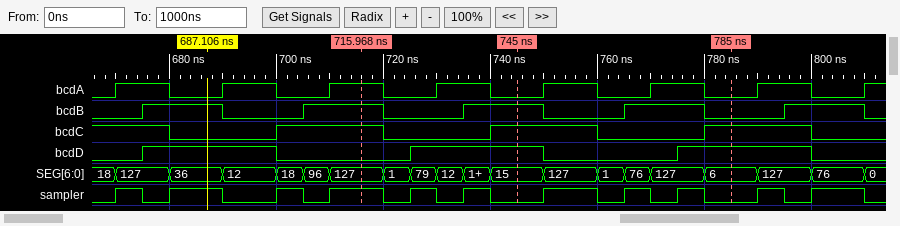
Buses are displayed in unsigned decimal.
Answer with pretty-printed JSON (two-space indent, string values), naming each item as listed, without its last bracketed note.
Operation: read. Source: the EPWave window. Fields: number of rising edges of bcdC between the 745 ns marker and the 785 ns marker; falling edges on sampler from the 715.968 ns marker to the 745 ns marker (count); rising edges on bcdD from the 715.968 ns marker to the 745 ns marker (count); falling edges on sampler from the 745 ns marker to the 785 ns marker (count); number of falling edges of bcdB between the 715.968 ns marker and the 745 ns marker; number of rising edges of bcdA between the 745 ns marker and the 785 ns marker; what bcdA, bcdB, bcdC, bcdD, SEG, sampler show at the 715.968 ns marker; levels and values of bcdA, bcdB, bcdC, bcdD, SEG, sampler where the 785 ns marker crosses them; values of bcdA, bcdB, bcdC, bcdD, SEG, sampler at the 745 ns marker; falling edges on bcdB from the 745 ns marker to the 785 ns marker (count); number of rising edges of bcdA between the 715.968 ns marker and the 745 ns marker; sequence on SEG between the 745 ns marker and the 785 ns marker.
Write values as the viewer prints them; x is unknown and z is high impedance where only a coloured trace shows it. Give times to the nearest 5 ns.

{
  "number of rising edges of bcdC between the 745 ns marker and the 785 ns marker": "1",
  "falling edges on sampler from the 715.968 ns marker to the 745 ns marker": "3",
  "rising edges on bcdD from the 715.968 ns marker to the 745 ns marker": "1",
  "falling edges on sampler from the 745 ns marker to the 785 ns marker": "3",
  "number of falling edges of bcdB between the 715.968 ns marker and the 745 ns marker": "1",
  "number of rising edges of bcdA between the 745 ns marker and the 785 ns marker": "2",
  "what bcdA, bcdB, bcdC, bcdD, SEG, sampler show at the 715.968 ns marker": "bcdA=1, bcdB=1, bcdC=1, bcdD=0, SEG=127, sampler=1",
  "levels and values of bcdA, bcdB, bcdC, bcdD, SEG, sampler where the 785 ns marker crosses them": "bcdA=0, bcdB=0, bcdC=1, bcdD=1, SEG=6, sampler=0",
  "values of bcdA, bcdB, bcdC, bcdD, SEG, sampler at the 745 ns marker": "bcdA=0, bcdB=1, bcdC=1, bcdD=1, SEG=15, sampler=0",
  "falling edges on bcdB from the 745 ns marker to the 785 ns marker": "2",
  "number of rising edges of bcdA between the 715.968 ns marker and the 745 ns marker": "1",
  "sequence on SEG between the 745 ns marker and the 785 ns marker": "15, 127, 1, 76, 127, 6"
}
